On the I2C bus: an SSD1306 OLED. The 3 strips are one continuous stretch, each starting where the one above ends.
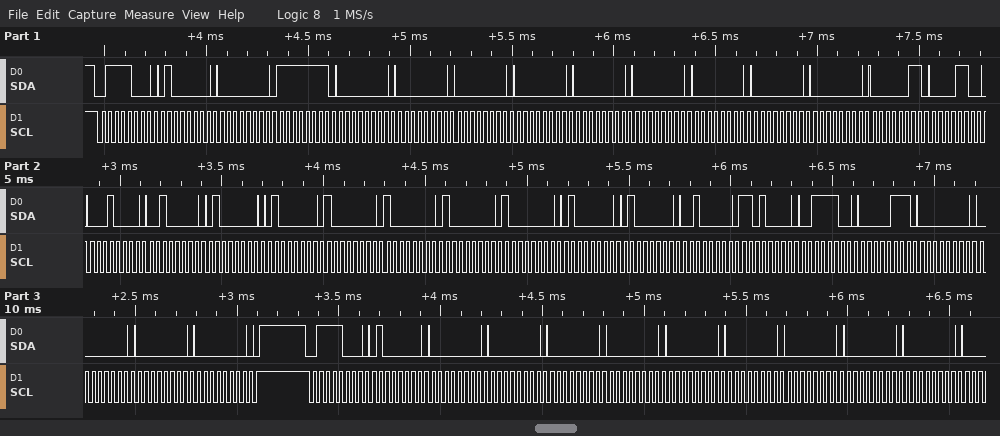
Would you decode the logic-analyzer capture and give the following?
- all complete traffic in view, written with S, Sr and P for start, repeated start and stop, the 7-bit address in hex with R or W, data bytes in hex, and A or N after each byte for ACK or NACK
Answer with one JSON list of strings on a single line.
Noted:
["S 3CW A 40 A 00 A FF A 00 A 00 A 00 A 00 A 00 A 00 A 00 A 00 A 00 A 03 A 0C A 10 A 20 A 40 A 40 A 80 A 80 A 80 A 80 A 40 A 40 A 20 A D0 A 3C A 07 A 00 A 00 A 00 A 00 A P S 3CW A 40 A 00 A 00 A 00 A 00 A 00 A 00 A 00 A 00 A 00 A"]
